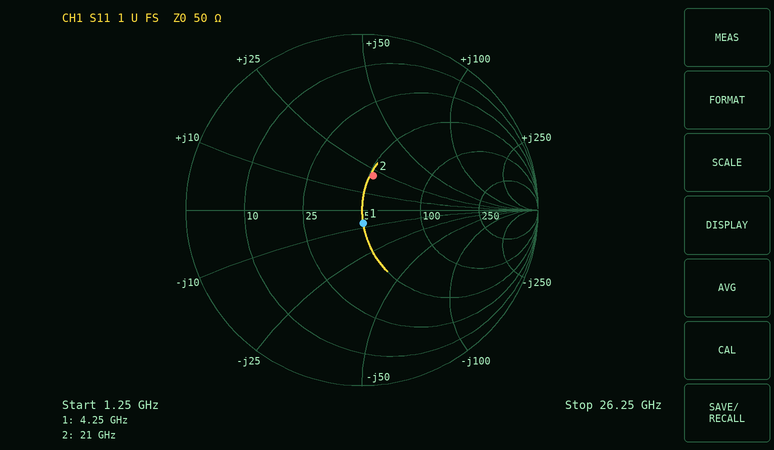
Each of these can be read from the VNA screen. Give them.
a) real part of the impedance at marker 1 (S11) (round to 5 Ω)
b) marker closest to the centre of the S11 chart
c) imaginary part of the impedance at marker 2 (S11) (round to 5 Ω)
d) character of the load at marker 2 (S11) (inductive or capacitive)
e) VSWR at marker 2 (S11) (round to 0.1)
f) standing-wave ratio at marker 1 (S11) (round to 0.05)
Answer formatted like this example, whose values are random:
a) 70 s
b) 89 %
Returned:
a) 50 Ω
b) marker 1
c) +20 Ω
d) inductive
e) 1.5
f) 1.15
